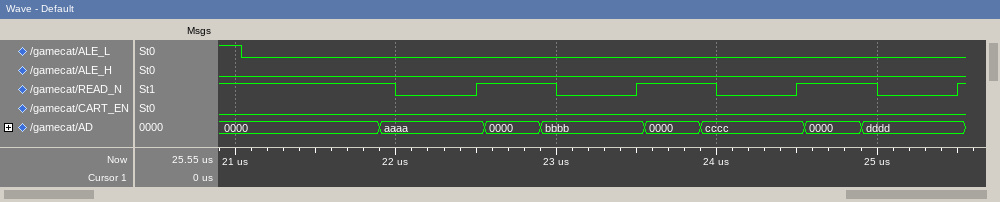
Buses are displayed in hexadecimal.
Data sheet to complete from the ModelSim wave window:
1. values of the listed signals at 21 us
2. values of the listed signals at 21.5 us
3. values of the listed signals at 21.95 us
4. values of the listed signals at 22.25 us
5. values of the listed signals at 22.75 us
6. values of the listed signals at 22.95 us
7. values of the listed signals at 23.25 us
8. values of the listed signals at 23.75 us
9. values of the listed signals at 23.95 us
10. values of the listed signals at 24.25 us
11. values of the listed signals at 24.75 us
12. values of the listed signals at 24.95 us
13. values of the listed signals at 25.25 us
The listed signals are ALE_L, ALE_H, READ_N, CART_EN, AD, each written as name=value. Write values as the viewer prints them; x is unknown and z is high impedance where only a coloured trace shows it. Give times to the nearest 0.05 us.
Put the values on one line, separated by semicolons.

ALE_L=1, ALE_H=0, READ_N=1, CART_EN=0, AD=0000; ALE_L=0, ALE_H=0, READ_N=1, CART_EN=0, AD=0000; ALE_L=0, ALE_H=0, READ_N=1, CART_EN=0, AD=aaaa; ALE_L=0, ALE_H=0, READ_N=0, CART_EN=0, AD=aaaa; ALE_L=0, ALE_H=0, READ_N=1, CART_EN=0, AD=0000; ALE_L=0, ALE_H=0, READ_N=1, CART_EN=0, AD=bbbb; ALE_L=0, ALE_H=0, READ_N=0, CART_EN=0, AD=bbbb; ALE_L=0, ALE_H=0, READ_N=1, CART_EN=0, AD=0000; ALE_L=0, ALE_H=0, READ_N=1, CART_EN=0, AD=cccc; ALE_L=0, ALE_H=0, READ_N=0, CART_EN=0, AD=cccc; ALE_L=0, ALE_H=0, READ_N=1, CART_EN=0, AD=0000; ALE_L=0, ALE_H=0, READ_N=1, CART_EN=0, AD=dddd; ALE_L=0, ALE_H=0, READ_N=0, CART_EN=0, AD=dddd
